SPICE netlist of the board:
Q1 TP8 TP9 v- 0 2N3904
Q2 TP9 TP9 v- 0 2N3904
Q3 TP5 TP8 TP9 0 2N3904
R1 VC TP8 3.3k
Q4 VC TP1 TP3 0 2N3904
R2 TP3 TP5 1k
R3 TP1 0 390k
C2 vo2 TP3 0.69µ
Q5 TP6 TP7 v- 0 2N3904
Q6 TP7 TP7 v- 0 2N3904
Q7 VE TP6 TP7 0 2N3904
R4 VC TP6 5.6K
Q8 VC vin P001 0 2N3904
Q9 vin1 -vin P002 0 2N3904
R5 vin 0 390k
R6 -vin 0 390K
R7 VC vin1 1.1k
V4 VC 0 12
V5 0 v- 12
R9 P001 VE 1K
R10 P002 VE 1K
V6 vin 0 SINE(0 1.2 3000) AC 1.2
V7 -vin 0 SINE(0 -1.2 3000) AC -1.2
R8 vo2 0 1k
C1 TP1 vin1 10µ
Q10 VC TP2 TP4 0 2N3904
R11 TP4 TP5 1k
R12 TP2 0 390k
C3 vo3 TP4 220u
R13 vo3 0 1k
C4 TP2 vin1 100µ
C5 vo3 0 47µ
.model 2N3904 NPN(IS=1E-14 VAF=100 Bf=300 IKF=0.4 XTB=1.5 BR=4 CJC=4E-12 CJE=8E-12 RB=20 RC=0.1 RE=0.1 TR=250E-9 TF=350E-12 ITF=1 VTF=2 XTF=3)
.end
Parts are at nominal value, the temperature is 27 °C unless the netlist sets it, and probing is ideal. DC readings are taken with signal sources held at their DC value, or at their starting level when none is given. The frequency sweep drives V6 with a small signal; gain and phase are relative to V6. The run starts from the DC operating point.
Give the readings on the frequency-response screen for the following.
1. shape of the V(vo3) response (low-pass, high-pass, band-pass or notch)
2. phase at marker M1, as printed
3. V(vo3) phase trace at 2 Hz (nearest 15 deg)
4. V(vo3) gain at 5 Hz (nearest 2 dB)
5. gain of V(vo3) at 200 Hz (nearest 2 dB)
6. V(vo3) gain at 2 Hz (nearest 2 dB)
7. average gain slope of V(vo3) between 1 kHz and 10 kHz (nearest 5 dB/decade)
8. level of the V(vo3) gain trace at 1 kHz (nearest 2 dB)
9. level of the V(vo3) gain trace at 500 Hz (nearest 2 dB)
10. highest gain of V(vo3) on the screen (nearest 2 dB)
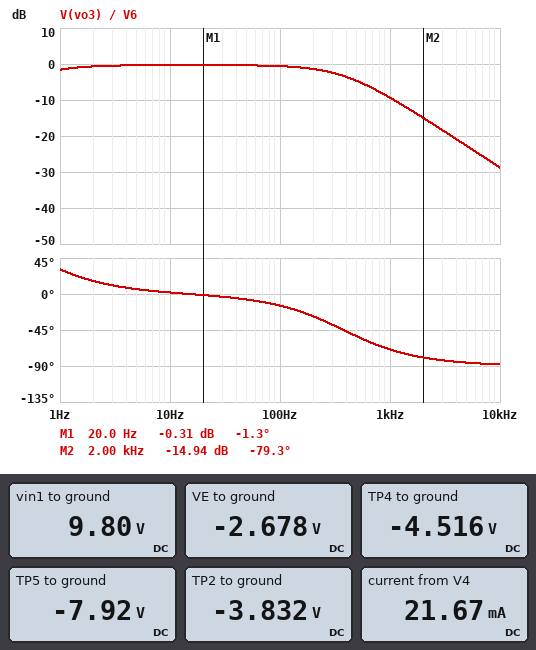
low-pass
-1.3 deg
15 deg
0 dB
-2 dB
0 dB
-20 dB/decade
-10 dB
-4 dB
0 dB
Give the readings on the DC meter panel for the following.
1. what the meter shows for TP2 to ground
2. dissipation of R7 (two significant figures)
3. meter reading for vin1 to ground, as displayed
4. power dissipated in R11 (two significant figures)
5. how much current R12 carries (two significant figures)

-3.832 V
4.4 mW
9.80 V
12 mW
9.8 µA
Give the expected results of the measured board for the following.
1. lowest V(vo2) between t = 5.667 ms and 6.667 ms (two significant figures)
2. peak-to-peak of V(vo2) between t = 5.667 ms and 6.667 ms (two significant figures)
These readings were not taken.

-1.2 V
2.4 V
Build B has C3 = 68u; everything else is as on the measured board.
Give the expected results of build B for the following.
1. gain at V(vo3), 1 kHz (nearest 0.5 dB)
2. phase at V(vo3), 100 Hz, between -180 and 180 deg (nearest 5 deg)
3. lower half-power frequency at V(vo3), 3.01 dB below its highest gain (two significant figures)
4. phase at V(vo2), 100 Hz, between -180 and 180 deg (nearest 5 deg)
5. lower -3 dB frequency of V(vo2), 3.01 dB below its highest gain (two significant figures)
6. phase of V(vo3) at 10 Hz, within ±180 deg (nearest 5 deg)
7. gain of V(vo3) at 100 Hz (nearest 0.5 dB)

-10.0 dB
-10 deg
1.4 Hz
65 deg
160 Hz
5 deg
-3.5 dB
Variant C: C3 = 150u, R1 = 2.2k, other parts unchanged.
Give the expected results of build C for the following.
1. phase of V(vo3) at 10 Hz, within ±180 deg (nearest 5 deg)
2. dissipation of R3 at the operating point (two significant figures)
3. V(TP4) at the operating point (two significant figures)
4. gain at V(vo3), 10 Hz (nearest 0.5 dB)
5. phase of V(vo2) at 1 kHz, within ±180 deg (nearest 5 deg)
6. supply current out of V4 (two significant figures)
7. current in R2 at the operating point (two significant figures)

5 deg
79 µW
-6.2 V
-1.0 dB
0 deg
28 mA
5.0 mA
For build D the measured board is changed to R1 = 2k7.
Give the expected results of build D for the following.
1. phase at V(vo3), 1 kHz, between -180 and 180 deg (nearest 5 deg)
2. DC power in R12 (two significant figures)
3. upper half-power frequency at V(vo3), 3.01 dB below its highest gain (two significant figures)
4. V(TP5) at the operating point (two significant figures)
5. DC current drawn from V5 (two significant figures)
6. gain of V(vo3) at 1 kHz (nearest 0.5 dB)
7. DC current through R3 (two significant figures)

-65 deg
56 µW
430 Hz
-9.5 V
25 mA
-8.5 dB
12 µA
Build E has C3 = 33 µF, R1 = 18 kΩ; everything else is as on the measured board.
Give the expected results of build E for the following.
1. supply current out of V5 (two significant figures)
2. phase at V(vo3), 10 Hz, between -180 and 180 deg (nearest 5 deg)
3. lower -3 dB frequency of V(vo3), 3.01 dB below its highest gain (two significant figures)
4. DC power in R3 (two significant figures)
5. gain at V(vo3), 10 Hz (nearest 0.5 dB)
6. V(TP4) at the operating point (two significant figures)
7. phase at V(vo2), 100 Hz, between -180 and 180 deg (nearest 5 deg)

11 mA
10 deg
1.9 Hz
1.3 µW
-6.5 dB
-1.4 V
65 deg
